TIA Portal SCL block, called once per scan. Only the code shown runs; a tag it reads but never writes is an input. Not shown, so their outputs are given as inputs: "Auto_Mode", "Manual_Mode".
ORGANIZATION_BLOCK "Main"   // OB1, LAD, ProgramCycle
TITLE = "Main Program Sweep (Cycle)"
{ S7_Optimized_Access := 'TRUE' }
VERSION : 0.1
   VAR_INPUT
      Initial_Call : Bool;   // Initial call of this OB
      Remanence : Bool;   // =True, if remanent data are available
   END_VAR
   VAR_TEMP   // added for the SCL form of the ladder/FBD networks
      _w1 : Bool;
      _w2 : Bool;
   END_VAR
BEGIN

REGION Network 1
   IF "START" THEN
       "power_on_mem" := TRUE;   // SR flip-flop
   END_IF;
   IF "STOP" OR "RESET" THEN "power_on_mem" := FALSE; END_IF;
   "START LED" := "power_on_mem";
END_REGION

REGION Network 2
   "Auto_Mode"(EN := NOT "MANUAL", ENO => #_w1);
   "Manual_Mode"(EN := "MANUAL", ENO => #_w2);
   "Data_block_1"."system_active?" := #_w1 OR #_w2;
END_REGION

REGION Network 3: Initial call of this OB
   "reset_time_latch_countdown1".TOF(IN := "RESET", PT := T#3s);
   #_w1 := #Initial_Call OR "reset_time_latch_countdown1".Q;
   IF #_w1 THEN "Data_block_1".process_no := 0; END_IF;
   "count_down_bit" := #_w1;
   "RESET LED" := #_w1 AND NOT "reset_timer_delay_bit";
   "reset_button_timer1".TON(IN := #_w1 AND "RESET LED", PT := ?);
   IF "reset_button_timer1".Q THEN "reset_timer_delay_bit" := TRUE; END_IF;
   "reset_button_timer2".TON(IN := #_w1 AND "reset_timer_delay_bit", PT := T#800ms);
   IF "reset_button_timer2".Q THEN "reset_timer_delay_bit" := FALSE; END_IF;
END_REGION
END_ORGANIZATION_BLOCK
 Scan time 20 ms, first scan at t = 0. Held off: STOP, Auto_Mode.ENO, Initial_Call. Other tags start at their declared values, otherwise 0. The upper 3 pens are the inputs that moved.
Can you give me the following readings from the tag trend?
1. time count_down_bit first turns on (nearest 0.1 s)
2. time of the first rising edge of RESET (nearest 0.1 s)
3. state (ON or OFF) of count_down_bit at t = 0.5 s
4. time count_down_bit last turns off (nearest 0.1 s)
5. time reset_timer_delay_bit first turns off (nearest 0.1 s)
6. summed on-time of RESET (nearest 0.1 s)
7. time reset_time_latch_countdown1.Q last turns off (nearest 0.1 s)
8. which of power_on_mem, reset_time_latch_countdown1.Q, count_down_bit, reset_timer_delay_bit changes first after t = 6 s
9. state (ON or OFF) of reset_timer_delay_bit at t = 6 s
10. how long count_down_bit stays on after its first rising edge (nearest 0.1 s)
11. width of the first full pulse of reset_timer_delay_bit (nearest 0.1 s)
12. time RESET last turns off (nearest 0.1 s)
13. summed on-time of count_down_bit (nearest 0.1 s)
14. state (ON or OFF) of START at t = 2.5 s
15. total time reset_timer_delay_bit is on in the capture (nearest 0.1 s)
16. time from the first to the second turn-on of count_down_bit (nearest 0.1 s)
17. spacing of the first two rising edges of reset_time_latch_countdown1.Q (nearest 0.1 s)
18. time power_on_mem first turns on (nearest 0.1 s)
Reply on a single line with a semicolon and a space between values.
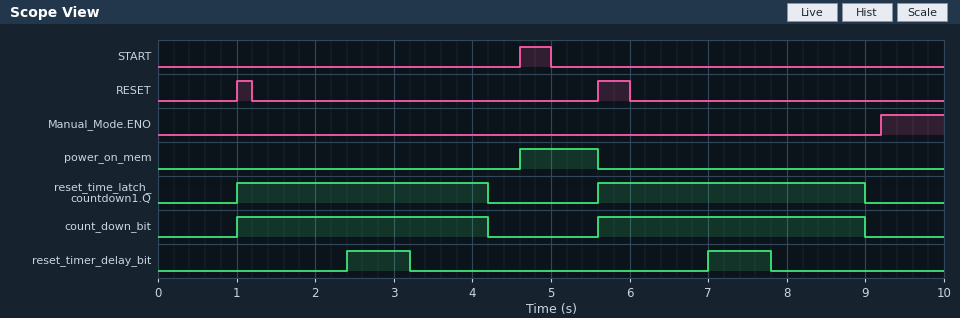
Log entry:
1.0 s; 1.0 s; OFF; 9.0 s; 3.2 s; 0.6 s; 9.0 s; reset_timer_delay_bit; OFF; 3.2 s; 0.8 s; 6.0 s; 6.6 s; OFF; 1.6 s; 4.6 s; 4.6 s; 4.6 s
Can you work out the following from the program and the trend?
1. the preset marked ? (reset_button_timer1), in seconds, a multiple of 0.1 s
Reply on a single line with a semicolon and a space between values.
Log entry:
1.4 s
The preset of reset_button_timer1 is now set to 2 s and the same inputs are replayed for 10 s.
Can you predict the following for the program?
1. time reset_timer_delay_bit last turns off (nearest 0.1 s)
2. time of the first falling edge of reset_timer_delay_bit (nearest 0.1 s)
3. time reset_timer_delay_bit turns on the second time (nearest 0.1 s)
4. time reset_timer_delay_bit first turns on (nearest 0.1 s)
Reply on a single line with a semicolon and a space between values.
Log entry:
8.4 s; 3.8 s; 7.6 s; 3.0 s
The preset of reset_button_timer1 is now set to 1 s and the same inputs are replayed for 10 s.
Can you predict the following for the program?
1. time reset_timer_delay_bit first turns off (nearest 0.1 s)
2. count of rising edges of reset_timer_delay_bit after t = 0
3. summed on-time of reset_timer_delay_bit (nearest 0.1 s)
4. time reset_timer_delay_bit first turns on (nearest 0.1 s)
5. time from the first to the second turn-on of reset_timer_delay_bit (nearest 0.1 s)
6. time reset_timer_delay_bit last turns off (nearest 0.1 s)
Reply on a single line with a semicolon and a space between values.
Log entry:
2.8 s; 3; 4.2 s; 2.0 s; 1.8 s; 8.2 s
